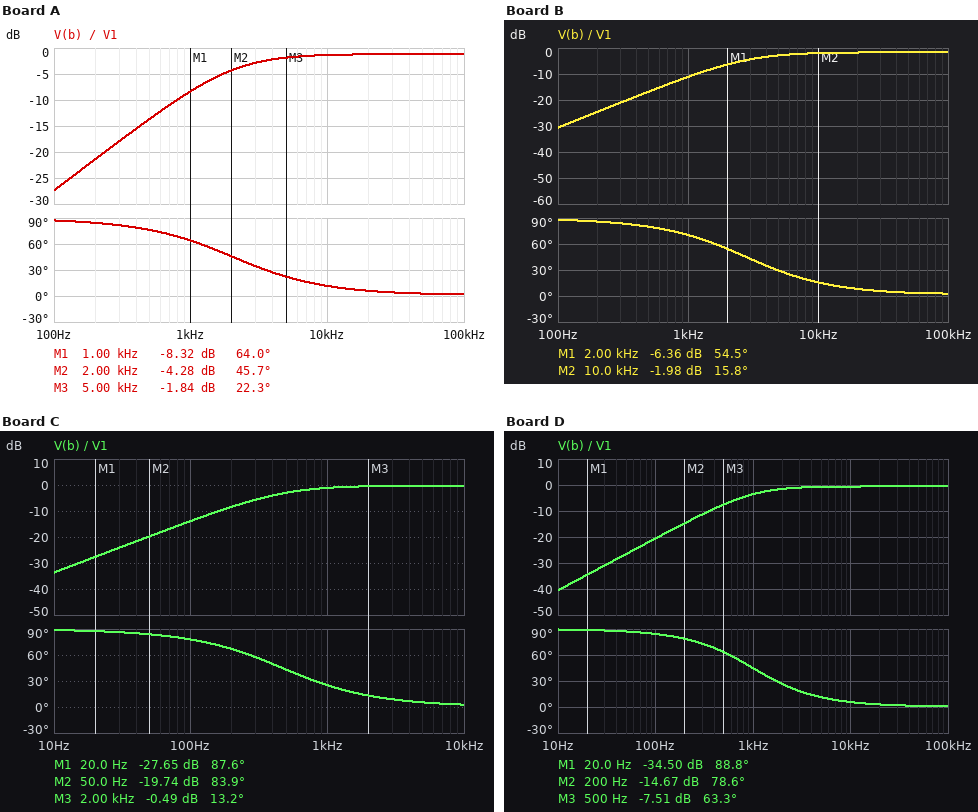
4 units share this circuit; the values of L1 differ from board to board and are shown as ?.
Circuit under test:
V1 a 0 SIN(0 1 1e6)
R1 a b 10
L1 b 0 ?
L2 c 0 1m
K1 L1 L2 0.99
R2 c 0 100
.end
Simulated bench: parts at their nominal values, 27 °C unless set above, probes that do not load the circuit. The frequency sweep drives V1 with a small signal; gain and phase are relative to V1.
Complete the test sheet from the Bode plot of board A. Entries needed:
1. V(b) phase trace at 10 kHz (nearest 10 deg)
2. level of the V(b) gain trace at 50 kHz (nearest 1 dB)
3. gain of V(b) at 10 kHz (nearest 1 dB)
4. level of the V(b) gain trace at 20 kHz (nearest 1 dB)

10 deg
-1 dB
-1 dB
-1 dB
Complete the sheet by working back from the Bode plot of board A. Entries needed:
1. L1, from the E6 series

680 µH
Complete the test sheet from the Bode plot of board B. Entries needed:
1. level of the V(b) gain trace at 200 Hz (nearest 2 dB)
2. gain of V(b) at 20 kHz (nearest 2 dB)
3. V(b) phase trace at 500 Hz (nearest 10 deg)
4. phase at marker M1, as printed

-24 dB
-2 dB
80 deg
54.5 deg
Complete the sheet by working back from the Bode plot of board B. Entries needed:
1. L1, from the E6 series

470 µH
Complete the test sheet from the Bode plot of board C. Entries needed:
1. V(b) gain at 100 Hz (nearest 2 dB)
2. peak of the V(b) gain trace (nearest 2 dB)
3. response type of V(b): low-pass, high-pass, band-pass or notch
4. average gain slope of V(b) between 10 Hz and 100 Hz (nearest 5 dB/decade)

-14 dB
0 dB
high-pass
20 dB/decade
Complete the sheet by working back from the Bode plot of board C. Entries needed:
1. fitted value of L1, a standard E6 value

3.3 mH
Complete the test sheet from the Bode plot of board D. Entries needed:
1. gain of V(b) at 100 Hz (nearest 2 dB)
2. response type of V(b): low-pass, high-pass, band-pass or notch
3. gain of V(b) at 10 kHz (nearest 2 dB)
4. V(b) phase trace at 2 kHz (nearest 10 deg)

-20 dB
high-pass
0 dB
30 deg
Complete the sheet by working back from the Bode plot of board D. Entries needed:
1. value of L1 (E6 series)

1.5 mH
